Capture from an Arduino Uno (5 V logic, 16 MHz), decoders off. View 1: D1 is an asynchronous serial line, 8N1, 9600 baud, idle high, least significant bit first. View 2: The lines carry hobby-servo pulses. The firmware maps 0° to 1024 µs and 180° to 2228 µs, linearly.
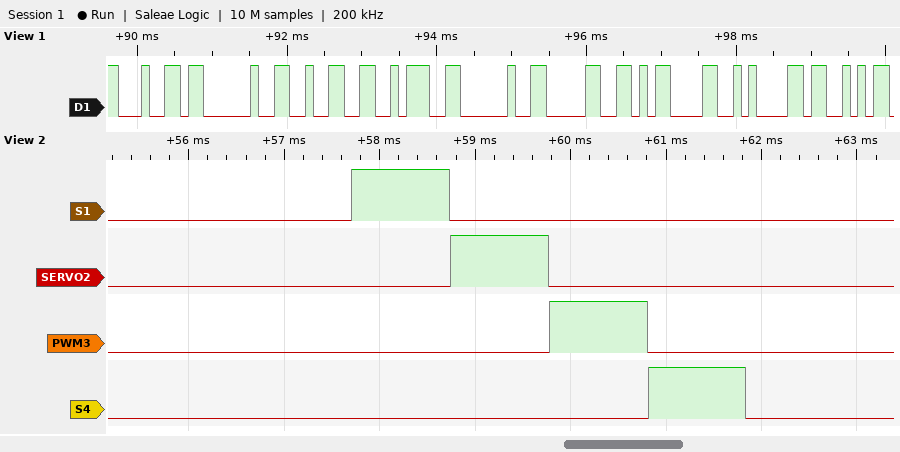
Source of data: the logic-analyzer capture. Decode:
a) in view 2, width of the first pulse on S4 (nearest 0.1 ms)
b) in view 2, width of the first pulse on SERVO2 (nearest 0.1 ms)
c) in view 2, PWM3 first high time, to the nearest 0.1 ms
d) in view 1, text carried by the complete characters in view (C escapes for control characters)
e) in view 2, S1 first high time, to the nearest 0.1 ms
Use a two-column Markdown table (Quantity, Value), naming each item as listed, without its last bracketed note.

| Quantity | Value |
|---|---|
| in view 2, width of the first pulse on S4 | 1.0 ms |
| in view 2, width of the first pulse on SERVO2 | 1.0 ms |
| in view 2, PWM3 first high time, to the nearest 0.1 ms | 1.0 ms |
| in view 1, text carried by the complete characters in view | "d 2: 0\r\nS" |
| in view 2, S1 first high time, to the nearest 0.1 ms | 1.0 ms |
